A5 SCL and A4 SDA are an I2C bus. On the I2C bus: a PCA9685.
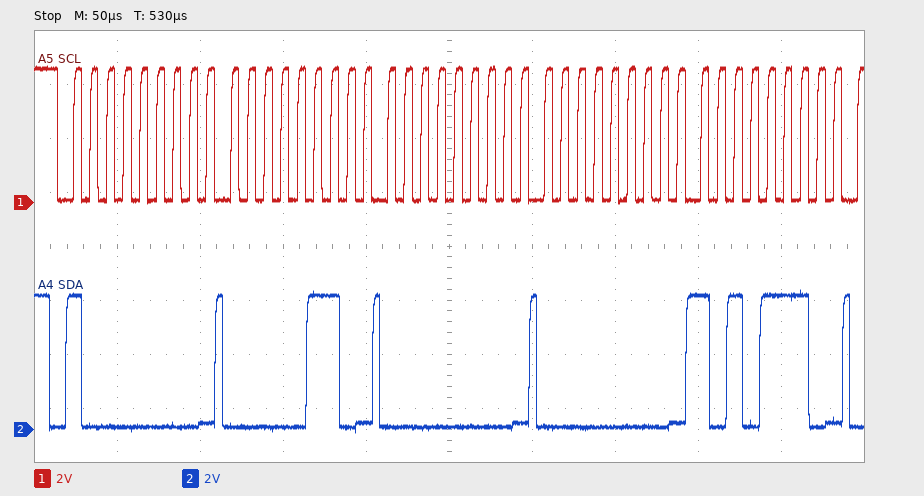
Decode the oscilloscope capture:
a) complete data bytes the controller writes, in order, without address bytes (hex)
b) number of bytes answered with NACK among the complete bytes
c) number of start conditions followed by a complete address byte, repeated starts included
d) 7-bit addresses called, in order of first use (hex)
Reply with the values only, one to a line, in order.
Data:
06 00 00 AE
0
1
0x40
